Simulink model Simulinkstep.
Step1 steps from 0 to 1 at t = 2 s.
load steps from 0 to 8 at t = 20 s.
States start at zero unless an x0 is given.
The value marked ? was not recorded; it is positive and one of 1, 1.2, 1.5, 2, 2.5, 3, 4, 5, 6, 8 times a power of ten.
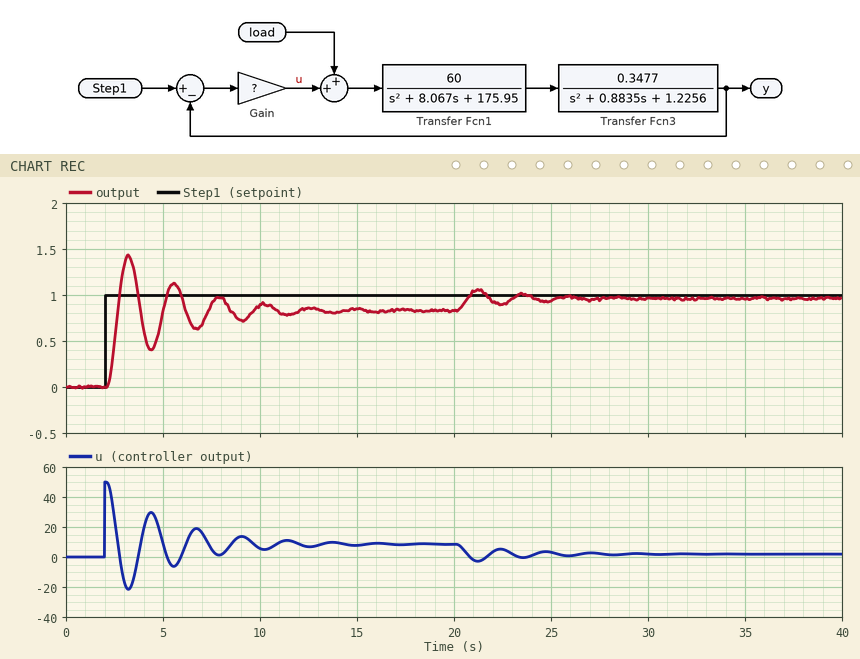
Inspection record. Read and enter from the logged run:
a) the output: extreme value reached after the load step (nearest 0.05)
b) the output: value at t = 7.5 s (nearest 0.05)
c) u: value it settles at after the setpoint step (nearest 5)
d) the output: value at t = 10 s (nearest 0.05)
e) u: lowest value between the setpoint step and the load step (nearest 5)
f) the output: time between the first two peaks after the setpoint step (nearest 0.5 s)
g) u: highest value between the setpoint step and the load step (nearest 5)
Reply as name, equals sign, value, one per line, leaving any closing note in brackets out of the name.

the output: extreme value reached after the load step = 1.05
the output: value at t = 7.5 s = 0.90
u: value it settles at after the setpoint step = 10
the output: value at t = 10 s = 0.90
u: lowest value between the setpoint step and the load step = -20
the output: time between the first two peaks after the setpoint step = 2.5 s
u: highest value between the setpoint step and the load step = 50
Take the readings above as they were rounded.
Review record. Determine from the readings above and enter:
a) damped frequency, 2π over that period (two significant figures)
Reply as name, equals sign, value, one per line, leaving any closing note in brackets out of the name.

damped frequency, 2π over that period = 2.5 rad/s
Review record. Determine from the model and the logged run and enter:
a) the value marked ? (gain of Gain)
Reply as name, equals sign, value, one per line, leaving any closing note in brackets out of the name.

the value marked ? = 50
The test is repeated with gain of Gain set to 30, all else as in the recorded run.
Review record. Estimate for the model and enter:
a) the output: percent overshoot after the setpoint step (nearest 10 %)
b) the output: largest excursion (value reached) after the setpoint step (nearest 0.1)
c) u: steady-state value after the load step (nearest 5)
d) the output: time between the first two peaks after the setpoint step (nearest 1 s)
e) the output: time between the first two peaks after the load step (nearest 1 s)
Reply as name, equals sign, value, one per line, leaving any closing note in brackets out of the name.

the output: percent overshoot after the setpoint step = 60 %
the output: largest excursion (value reached) after the setpoint step = 1.2
u: steady-state value after the load step = 0
the output: time between the first two peaks after the setpoint step = 3 s
the output: time between the first two peaks after the load step = 3 s
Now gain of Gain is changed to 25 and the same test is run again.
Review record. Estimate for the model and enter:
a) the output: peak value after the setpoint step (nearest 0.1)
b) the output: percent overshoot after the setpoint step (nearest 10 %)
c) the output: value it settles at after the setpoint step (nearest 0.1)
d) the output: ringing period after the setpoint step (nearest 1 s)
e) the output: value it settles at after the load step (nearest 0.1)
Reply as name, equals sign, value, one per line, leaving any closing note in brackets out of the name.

the output: peak value after the setpoint step = 1.1
the output: percent overshoot after the setpoint step = 60 %
the output: value it settles at after the setpoint step = 0.7
the output: ringing period after the setpoint step = 3 s
the output: value it settles at after the load step = 0.9
